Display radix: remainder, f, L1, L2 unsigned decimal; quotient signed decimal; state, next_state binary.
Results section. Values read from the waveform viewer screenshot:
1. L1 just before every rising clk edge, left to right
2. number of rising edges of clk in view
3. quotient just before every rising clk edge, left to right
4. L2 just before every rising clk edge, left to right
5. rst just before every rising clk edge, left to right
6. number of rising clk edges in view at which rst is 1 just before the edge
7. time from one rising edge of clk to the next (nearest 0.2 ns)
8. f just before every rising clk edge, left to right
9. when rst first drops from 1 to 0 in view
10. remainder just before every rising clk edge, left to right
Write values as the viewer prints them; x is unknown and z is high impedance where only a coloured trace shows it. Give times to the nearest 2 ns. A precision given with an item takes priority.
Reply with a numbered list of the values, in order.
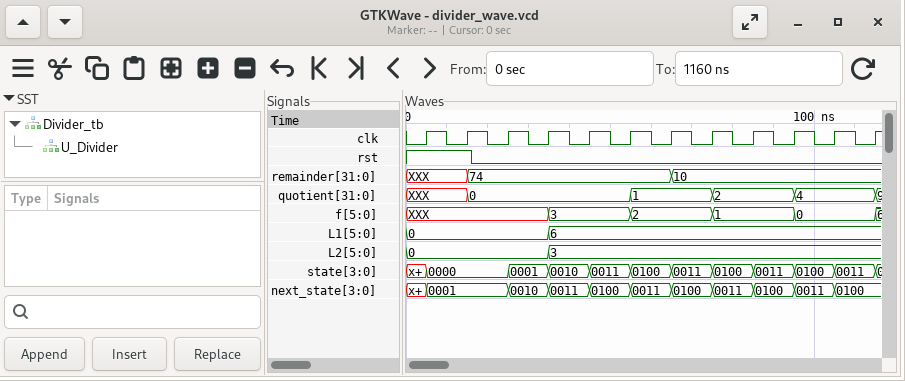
1. 0, 0, 0, 0, 6, 6, 6, 6, 6, 6, 6, 6
2. 12
3. XXX, XXX, 0, 0, 0, 0, 1, 1, 2, 2, 4, 4
4. 0, 0, 0, 0, 3, 3, 3, 3, 3, 3, 3, 3
5. 1 1 0 0 0 0 0 0 0 0 0 0
6. 2
7. 10 ns
8. XXX, XXX, XXX, XXX, 3, 3, 2, 2, 1, 1, 0, 0
9. 16 ns
10. XXX, XXX, 74, 74, 74, 74, 74, 10, 10, 10, 10, 10
